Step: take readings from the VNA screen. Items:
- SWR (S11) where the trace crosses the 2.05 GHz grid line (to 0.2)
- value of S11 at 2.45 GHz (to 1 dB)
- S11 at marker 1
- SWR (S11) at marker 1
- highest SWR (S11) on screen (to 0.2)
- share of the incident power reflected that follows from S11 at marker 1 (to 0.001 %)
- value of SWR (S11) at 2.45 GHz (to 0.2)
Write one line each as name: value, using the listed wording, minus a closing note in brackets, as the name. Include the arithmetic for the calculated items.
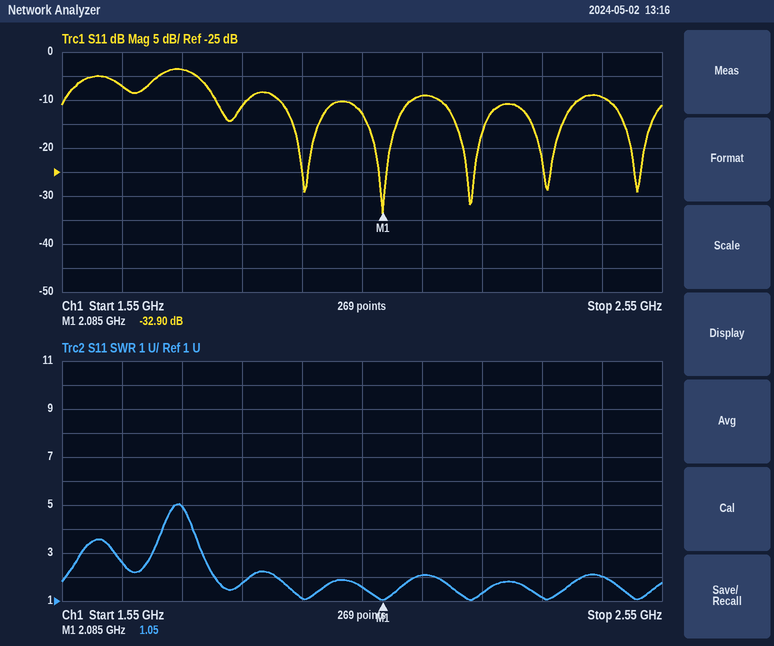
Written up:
SWR (S11) where the trace crosses the 2.05 GHz grid line: 1.6
value of S11 at 2.45 GHz: -9 dB
S11 at marker 1: -32.90 dB
SWR (S11) at marker 1: 1.05
highest SWR (S11) on screen: 5.0
share of the incident power reflected that follows from S11 at marker 1: 10^(-32.9/10) ≈ 0.051 %
value of SWR (S11) at 2.45 GHz: 2.0
